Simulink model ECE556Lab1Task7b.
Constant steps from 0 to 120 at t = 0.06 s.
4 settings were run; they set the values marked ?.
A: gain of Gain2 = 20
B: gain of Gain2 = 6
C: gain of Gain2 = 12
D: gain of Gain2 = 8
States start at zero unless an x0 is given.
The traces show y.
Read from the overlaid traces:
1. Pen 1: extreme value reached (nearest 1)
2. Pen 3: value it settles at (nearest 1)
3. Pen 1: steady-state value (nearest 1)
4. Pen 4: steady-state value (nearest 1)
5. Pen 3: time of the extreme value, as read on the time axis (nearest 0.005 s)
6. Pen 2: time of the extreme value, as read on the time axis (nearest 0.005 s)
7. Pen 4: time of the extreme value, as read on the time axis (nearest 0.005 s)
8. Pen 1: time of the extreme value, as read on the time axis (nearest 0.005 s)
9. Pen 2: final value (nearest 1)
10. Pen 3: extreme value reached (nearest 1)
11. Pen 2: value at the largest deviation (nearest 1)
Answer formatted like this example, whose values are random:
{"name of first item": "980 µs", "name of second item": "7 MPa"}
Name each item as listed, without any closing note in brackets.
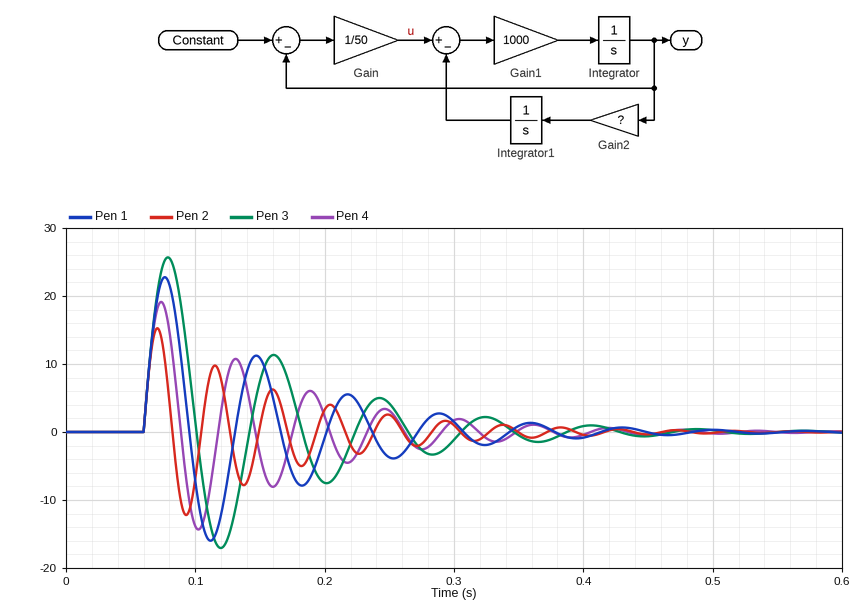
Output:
{"Pen 1: extreme value reached": "23", "Pen 3: value it settles at": "0", "Pen 1: steady-state value": "0", "Pen 4: steady-state value": "0", "Pen 3: time of the extreme value, as read on the time axis": "0.080 s", "Pen 2: time of the extreme value, as read on the time axis": "0.070 s", "Pen 4: time of the extreme value, as read on the time axis": "0.075 s", "Pen 1: time of the extreme value, as read on the time axis": "0.075 s", "Pen 2: final value": "0", "Pen 3: extreme value reached": "26", "Pen 2: value at the largest deviation": "15"}
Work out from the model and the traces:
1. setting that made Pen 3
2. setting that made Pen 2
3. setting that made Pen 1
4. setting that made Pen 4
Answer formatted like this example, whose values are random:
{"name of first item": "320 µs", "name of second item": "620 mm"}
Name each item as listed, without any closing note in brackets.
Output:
{"setting that made Pen 3": "B", "setting that made Pen 2": "A", "setting that made Pen 1": "D", "setting that made Pen 4": "C"}
